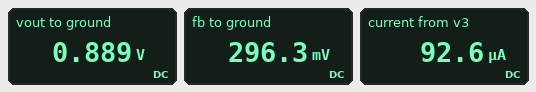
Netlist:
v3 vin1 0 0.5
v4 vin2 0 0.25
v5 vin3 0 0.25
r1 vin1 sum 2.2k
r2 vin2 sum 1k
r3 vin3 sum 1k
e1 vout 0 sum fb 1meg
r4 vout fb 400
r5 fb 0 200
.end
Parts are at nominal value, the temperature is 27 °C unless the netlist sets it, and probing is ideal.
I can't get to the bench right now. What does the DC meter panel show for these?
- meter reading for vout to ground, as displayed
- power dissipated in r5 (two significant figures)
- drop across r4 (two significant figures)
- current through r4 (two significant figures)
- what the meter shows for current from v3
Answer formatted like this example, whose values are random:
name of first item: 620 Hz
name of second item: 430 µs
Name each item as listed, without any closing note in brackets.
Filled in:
meter reading for vout to ground, as displayed: 0.889 V
power dissipated in r5: 440 µW
drop across r4: 590 mV
current through r4: 1.5 mA
what the meter shows for current from v3: 92.6 µA
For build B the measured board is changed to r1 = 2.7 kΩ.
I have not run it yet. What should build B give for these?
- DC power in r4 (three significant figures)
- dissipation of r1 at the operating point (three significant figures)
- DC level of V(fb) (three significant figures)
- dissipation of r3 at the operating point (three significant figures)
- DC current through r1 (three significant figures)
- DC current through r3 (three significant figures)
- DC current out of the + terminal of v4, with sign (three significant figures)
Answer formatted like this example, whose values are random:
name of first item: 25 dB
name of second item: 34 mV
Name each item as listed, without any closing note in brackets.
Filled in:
DC power in r4: 836 µW
dissipation of r1 at the operating point: 16.5 µW
DC level of V(fb): 289 mV
dissipation of r3 at the operating point: 1.53 µW
DC current through r1: 78.1 µA
DC current through r3: 39.1 µA
DC current out of the + terminal of v4, with sign: -39.1 µA
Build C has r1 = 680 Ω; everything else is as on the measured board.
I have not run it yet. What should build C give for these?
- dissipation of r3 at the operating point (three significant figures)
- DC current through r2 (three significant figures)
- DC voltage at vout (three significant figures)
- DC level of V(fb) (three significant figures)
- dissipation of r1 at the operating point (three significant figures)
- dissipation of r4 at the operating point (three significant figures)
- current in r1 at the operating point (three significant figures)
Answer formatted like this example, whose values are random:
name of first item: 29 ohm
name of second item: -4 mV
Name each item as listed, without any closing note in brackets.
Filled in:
dissipation of r3 at the operating point: 11.2 µW
DC current through r2: 106 µA
DC voltage at vout: 1.07 V
DC level of V(fb): 356 mV
dissipation of r1 at the operating point: 30.5 µW
dissipation of r4 at the operating point: 1.27 mW
current in r1 at the operating point: 212 µA
